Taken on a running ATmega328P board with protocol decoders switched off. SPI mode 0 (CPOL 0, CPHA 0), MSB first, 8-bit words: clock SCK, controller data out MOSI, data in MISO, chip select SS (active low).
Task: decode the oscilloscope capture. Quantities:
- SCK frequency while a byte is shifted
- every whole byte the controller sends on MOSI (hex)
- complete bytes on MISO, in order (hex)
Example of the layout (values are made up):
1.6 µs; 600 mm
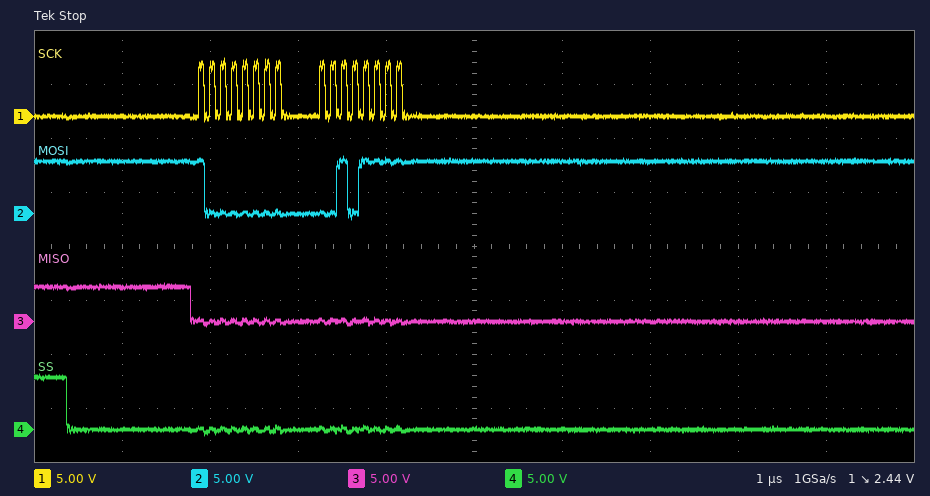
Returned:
8 MHz; 80 2F; 00 00
